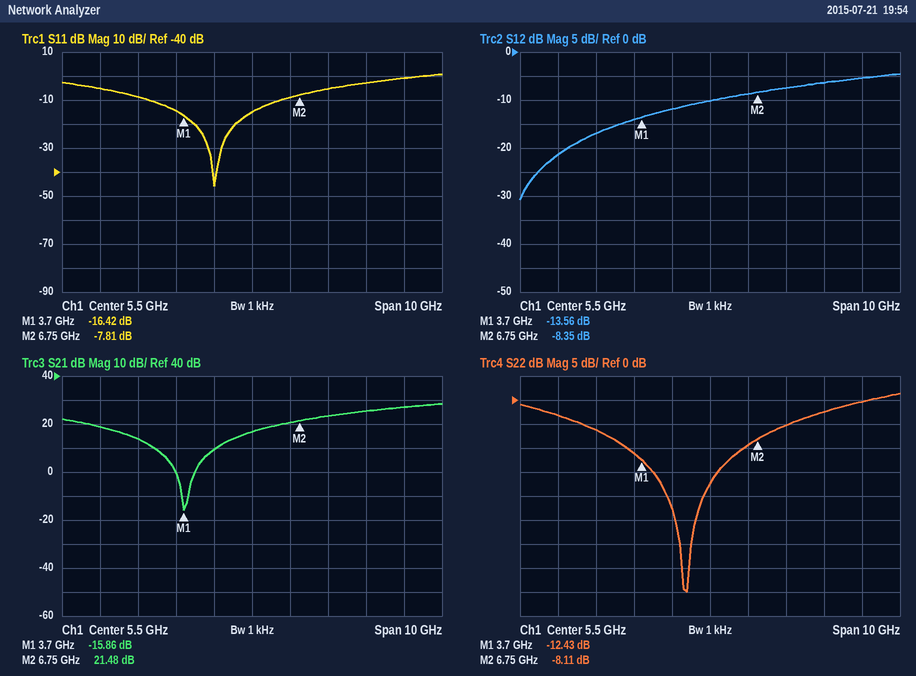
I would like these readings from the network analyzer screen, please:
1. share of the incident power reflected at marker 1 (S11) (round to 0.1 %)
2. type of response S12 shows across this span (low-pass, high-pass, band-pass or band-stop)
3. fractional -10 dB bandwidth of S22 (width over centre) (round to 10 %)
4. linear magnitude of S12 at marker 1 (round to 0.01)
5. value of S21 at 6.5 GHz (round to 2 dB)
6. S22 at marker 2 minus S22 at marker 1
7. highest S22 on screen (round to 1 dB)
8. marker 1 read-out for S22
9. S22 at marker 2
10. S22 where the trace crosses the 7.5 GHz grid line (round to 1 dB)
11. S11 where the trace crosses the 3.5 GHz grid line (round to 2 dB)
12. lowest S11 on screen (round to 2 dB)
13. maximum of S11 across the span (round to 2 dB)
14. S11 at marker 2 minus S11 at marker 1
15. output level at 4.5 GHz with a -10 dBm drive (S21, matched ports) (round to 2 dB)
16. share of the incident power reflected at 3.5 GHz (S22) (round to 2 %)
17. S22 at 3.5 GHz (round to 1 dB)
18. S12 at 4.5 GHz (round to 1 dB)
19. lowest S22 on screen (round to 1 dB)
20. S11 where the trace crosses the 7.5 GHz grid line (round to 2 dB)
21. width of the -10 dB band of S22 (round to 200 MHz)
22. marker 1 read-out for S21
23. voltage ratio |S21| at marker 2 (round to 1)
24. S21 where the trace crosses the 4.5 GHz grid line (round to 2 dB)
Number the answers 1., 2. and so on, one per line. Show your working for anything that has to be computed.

1. 10^(-16.42/10) ≈ 2.3 %
2. high-pass
3. 3 GHz / 4.9 GHz ≈ 61.2 %, so 60 % to the nearest 10 %
4. 10^(-13.56/20) ≈ 0.21
5. 20 dB
6. -8.11 − (-12.43) = 4.32 dB
7. 1 dB
8. -12.43 dB
9. -8.11 dB
10. -5 dB
11. -14 dB
12. -46 dB
13. 0 dB
14. -7.81 − (-16.42) = 8.61 dB
15. -10 dBm + (10 dB) = 0 dBm
16. 10^(-11/10) ≈ 8 %
17. -11 dB
18. -12 dB
19. -40 dB
20. -6 dB
21. 6.4 GHz − 3.4 GHz = 3.0 GHz
22. -15.86 dB
23. 10^(21.48/20) ≈ 12
24. 10 dB
